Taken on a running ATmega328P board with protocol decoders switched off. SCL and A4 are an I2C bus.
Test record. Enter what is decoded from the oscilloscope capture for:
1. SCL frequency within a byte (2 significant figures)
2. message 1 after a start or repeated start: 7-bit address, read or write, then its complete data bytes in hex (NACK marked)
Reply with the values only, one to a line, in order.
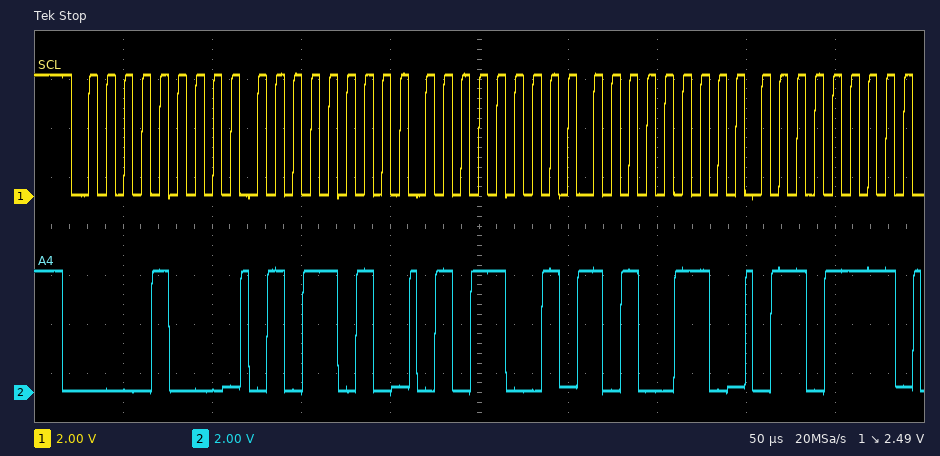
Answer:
100 kHz
0x04 write: 5A 59 A6 6F
